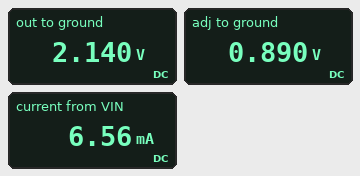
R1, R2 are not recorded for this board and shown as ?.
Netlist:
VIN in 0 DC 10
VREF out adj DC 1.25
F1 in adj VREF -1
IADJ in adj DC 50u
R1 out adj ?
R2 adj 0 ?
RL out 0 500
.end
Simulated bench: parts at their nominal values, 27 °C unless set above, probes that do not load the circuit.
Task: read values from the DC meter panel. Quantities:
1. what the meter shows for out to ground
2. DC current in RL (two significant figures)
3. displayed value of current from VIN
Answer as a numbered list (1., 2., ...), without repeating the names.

1. 2.140 V
2. 4.3 mA
3. 6.56 mA
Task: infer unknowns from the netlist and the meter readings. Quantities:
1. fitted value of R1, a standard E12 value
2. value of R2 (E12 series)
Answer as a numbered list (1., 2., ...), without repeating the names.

1. 560 Ω
2. 390 Ω
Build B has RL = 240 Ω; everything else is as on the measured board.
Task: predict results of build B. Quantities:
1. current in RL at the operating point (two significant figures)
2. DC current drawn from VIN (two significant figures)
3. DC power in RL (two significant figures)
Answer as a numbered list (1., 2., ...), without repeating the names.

1. 8.9 mA
2. 11 mA
3. 19 mW
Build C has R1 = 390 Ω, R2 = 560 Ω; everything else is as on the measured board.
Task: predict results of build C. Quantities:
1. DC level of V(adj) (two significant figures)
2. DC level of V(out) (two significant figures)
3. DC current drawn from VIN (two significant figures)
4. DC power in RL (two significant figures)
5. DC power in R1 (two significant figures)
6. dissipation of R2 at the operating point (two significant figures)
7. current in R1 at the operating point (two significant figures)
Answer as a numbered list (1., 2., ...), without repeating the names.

1. 1.8 V
2. 3.1 V
3. 9.4 mA
4. 19 mW
5. 4.0 mW
6. 5.9 mW
7. 3.2 mA
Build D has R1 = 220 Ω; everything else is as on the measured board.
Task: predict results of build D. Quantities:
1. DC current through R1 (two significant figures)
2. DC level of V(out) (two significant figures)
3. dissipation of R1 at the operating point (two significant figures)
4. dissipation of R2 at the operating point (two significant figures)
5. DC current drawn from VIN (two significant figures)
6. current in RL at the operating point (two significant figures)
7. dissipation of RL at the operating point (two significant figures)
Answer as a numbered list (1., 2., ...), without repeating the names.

1. 5.7 mA
2. 3.5 V
3. 7.1 mW
4. 13 mW
5. 13 mA
6. 7.0 mA
7. 24 mW
